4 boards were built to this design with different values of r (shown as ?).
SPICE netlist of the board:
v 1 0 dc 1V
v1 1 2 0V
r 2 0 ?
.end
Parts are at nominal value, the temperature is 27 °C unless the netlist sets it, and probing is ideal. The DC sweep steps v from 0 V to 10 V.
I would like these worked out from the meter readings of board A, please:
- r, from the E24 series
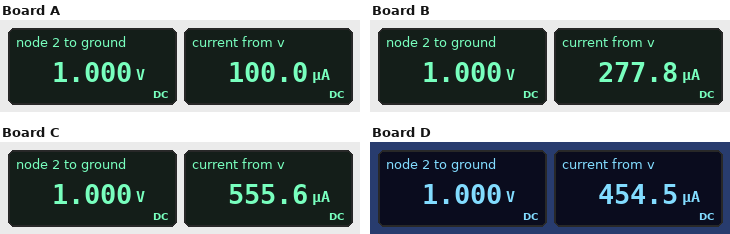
10 kΩ
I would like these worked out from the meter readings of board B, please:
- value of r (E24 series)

3.6 kΩ
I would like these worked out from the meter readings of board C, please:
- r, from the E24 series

1.8 kΩ
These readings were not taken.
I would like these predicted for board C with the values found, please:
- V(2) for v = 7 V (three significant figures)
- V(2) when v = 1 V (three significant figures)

7.00 V
1.00 V
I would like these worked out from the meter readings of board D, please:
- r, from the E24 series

2.2 kΩ
